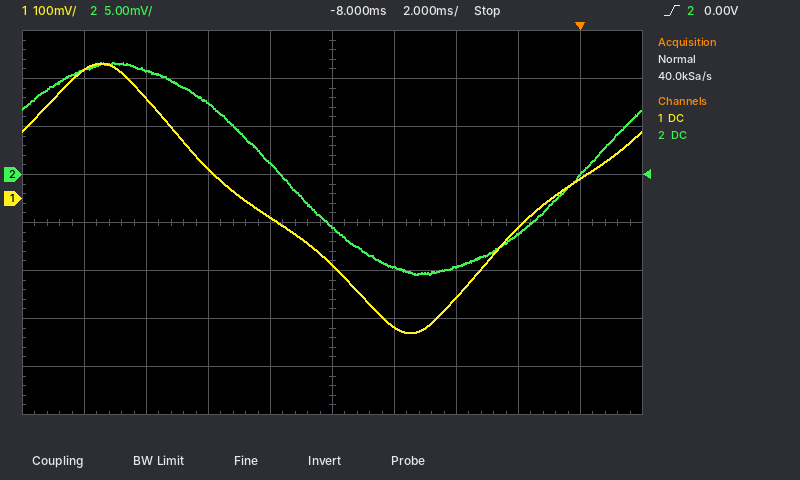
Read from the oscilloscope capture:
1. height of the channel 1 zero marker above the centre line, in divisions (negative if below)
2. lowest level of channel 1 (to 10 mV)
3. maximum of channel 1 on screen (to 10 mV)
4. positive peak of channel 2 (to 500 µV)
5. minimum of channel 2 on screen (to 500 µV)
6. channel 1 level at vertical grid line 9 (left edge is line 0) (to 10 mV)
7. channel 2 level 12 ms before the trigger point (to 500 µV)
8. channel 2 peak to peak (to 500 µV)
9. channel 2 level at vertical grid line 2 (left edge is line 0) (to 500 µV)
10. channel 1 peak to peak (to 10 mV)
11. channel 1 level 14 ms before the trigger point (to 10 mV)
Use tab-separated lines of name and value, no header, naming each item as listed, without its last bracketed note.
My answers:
height of the channel 1 zero marker above the centre line, in divisions	+0.5 div
lowest level of channel 1	-280 mV
maximum of channel 1 on screen	280 mV
positive peak of channel 2	11.5 mV
minimum of channel 2 on screen	-10.5 mV
channel 1 level at vertical grid line 9 (left edge is line 0)	40 mV
channel 2 level 12 ms before the trigger point	7.5 mV
channel 2 peak to peak	22.0 mV
channel 2 level at vertical grid line 2 (left edge is line 0)	11.0 mV
channel 1 peak to peak	560 mV
channel 1 level 14 ms before the trigger point	210 mV
